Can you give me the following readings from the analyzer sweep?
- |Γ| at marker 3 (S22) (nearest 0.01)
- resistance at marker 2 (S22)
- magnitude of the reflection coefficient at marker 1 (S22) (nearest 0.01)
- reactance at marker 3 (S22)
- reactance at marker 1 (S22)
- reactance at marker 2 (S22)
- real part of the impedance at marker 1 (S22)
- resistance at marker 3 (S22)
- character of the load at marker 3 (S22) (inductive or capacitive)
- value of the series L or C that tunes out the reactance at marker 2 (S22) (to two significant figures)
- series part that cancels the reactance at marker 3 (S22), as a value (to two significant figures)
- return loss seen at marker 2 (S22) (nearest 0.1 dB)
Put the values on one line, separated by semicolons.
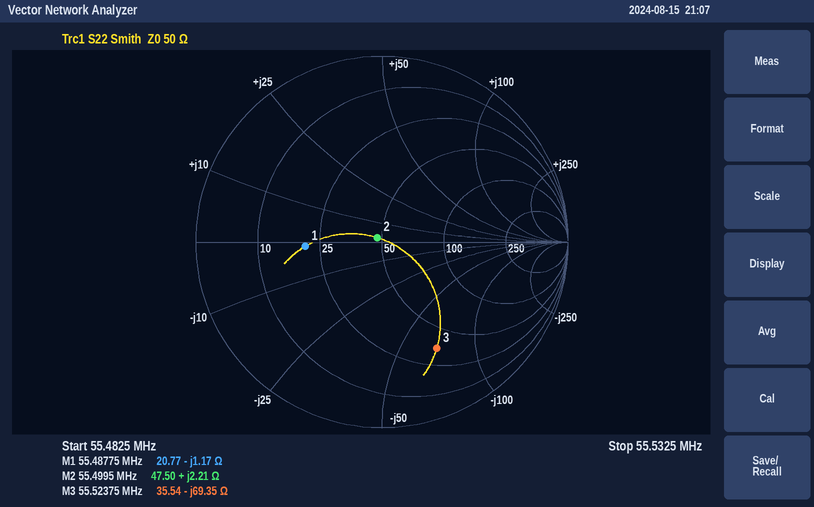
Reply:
0.64; 47.50 Ω; 0.41; -69.35 Ω; -1.17 Ω; +2.21 Ω; 20.77 Ω; 35.54 Ω; capacitive; 1.3 nF; 200 nH; 29.3 dB
